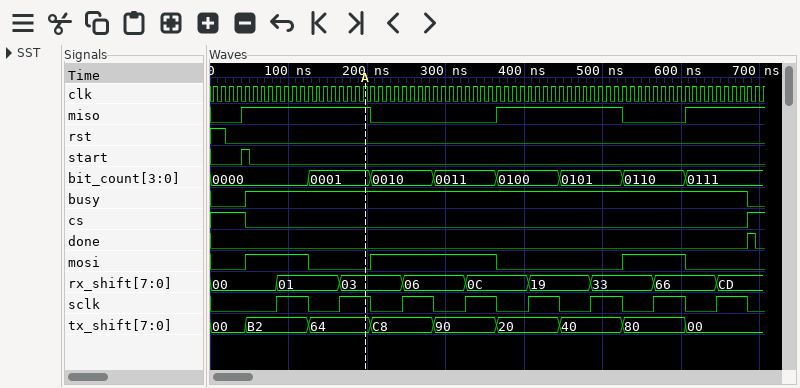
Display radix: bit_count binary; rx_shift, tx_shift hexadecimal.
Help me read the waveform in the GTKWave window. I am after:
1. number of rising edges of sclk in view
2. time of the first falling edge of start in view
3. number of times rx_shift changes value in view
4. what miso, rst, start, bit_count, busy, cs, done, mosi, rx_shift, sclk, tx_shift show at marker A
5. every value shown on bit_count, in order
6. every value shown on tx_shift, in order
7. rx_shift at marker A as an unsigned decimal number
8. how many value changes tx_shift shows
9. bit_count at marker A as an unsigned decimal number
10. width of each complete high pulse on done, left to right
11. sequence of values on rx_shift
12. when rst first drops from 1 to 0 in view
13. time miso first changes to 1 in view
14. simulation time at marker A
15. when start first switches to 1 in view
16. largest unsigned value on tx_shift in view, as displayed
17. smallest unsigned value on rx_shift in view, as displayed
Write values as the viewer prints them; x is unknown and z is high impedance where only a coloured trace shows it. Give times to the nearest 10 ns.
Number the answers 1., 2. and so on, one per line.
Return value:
1. 8
2. 50 ns
3. 8
4. miso=1, rst=0, start=0, bit_count=0001, busy=1, cs=0, done=0, mosi=0, rx_shift=03, sclk=1, tx_shift=64
5. 0000, 0001, 0010, 0011, 0100, 0101, 0110, 0111
6. 00, B2, 64, C8, 90, 20, 40, 80, 00
7. 3
8. 8
9. 1
10. 10 ns
11. 00, 01, 03, 06, 0C, 19, 33, 66, CD
12. 20 ns
13. 40 ns
14. 200 ns
15. 40 ns
16. C8
17. 00
